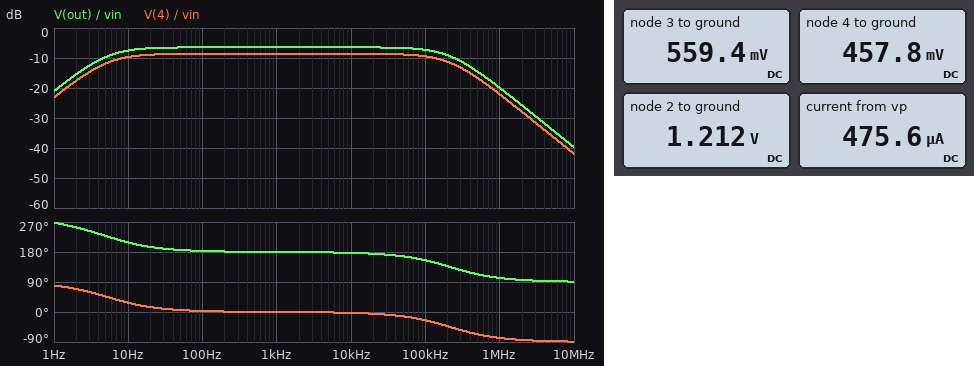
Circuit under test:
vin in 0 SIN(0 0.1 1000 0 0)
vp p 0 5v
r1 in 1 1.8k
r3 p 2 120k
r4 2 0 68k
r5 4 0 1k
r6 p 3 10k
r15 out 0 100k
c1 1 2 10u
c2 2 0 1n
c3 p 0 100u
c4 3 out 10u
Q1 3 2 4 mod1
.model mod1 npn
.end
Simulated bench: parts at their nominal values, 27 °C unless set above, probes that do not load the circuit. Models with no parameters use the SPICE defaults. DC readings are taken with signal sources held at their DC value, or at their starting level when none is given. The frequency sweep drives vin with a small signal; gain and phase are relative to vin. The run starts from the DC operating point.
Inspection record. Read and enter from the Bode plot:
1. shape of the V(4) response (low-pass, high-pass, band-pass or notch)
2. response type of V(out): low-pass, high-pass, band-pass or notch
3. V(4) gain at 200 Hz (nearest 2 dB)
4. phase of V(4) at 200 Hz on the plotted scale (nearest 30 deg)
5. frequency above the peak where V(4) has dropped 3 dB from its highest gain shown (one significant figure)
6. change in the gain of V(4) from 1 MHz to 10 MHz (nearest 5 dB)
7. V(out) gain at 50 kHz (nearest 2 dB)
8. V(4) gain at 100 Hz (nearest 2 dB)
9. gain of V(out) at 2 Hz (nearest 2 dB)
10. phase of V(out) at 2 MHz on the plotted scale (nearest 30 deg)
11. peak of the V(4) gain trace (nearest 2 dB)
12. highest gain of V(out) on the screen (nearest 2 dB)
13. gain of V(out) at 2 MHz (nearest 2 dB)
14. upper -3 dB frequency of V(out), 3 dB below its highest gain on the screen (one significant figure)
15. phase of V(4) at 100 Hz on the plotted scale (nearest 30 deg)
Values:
band-pass
band-pass
-8 dB
0 deg
200 kHz
-20 dB
-6 dB
-8 dB
-16 dB
90 deg
-8 dB
-6 dB
-26 dB
200 kHz
0 deg
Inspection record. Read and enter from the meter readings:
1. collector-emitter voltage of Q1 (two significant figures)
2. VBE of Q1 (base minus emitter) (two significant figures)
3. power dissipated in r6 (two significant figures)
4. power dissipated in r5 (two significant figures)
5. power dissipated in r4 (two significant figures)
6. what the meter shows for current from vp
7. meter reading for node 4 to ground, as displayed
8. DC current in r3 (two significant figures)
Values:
100 mV
750 mV
2.0 mW
210 µW
22 µW
475.6 µA
457.8 mV
32 µA
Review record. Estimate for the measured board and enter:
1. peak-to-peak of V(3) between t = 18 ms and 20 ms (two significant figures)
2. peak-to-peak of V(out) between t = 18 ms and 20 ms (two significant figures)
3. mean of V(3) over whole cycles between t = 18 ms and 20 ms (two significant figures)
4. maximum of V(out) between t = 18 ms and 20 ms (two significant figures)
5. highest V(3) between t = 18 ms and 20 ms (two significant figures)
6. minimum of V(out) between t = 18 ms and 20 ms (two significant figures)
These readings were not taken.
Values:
670 mV
670 mV
750 mV
660 mV
1.2 V
-11 mV
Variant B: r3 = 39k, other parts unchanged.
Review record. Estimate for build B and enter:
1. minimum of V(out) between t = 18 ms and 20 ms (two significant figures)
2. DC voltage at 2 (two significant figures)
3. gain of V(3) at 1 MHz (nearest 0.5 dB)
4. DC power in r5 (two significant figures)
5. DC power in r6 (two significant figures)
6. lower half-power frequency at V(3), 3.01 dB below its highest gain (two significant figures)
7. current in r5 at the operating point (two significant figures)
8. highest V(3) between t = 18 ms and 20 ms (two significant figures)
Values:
-19 mV
1.3 V
-25.0 dB
270 µW
2.0 mW
5.7 Hz
520 µA
600 mV
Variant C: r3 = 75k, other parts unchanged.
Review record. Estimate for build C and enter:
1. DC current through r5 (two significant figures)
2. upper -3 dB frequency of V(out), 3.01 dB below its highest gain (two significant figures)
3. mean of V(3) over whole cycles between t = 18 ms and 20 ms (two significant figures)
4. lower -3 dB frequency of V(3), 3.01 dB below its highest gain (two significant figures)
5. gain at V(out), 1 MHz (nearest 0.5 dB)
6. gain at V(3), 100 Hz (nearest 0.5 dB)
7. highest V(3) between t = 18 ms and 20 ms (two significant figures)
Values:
480 µA
240 kHz
580 mV
5.6 Hz
-38.5 dB
-26.0 dB
710 mV
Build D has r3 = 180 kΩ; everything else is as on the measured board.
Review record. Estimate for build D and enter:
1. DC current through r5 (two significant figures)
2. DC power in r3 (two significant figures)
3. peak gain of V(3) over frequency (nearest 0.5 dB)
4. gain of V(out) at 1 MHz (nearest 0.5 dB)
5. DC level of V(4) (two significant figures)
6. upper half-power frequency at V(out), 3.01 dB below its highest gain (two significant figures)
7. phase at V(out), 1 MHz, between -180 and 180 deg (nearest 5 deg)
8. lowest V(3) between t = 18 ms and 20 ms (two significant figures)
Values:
420 µA
82 µW
18.0 dB
-2.5 dB
420 mV
93 kHz
95 deg
560 mV
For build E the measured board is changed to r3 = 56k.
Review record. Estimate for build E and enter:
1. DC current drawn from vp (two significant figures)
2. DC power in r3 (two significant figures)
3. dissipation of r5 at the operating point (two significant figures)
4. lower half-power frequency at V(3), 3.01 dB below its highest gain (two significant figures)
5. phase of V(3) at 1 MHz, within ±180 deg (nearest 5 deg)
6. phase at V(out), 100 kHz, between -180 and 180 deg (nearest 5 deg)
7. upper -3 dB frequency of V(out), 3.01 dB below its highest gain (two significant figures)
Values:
510 µA
250 µW
240 µW
5.7 Hz
-75 deg
-20 deg
250 kHz
